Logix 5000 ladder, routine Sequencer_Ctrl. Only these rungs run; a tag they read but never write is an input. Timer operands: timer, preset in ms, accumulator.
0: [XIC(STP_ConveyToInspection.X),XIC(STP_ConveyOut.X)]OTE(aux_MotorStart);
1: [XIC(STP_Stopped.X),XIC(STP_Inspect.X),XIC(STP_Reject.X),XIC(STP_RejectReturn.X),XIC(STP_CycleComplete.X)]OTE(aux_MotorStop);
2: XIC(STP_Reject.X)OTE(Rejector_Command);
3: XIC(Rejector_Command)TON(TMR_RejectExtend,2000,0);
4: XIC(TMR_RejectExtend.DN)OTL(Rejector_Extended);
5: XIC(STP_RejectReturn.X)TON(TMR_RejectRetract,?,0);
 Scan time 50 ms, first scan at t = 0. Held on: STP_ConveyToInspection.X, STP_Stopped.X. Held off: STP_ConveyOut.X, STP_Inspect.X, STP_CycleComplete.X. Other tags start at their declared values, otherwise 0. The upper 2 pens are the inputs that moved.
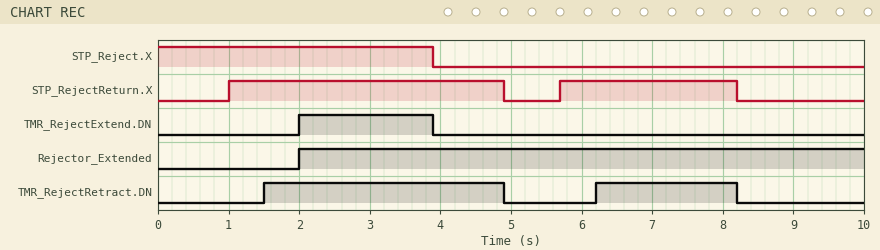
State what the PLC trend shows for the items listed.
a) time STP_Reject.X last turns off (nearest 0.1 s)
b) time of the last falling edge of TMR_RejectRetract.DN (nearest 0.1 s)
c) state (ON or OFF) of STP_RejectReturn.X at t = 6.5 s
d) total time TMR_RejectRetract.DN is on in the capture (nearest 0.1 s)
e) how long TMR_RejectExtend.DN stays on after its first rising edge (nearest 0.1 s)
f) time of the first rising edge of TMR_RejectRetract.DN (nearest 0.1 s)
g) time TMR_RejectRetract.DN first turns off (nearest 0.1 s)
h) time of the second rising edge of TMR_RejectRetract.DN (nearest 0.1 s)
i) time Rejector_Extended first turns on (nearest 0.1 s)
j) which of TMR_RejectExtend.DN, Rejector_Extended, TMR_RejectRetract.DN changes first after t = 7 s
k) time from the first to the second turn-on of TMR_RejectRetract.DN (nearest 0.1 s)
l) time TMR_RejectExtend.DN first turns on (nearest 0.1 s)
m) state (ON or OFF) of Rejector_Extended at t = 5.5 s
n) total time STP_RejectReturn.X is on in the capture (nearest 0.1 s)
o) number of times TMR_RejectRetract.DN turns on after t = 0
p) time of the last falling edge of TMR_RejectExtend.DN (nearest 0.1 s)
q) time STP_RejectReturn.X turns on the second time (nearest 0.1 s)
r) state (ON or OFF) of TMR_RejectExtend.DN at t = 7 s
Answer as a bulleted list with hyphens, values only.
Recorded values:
- 3.9 s
- 8.2 s
- ON
- 5.4 s
- 1.9 s
- 1.5 s
- 4.9 s
- 6.2 s
- 2.0 s
- TMR_RejectRetract.DN
- 4.7 s
- 2.0 s
- ON
- 6.4 s
- 2
- 3.9 s
- 5.7 s
- OFF
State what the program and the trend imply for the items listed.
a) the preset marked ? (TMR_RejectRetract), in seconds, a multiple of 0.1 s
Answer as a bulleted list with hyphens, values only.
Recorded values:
- 0.5 s
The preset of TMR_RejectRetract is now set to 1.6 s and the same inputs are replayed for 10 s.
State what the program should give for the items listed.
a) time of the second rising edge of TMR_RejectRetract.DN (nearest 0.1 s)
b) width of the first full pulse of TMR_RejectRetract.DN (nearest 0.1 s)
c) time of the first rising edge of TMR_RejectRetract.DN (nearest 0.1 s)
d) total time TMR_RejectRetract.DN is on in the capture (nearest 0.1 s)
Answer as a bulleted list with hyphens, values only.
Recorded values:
- 7.3 s
- 2.3 s
- 2.6 s
- 3.2 s
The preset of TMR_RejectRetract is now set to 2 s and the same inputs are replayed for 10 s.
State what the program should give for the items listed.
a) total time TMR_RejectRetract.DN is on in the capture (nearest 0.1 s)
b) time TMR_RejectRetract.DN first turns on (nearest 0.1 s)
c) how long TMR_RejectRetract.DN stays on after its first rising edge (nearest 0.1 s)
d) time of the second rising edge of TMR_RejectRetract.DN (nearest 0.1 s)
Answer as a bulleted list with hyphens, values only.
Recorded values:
- 2.4 s
- 3.0 s
- 1.9 s
- 7.7 s
